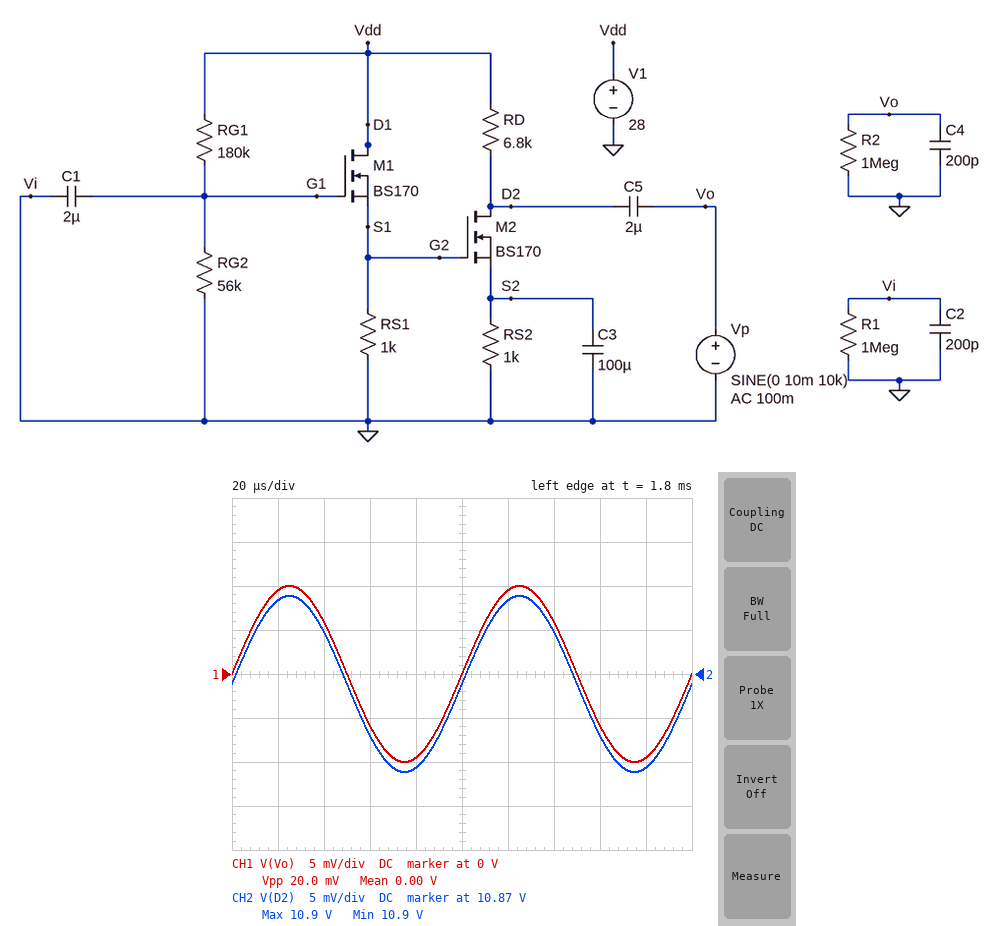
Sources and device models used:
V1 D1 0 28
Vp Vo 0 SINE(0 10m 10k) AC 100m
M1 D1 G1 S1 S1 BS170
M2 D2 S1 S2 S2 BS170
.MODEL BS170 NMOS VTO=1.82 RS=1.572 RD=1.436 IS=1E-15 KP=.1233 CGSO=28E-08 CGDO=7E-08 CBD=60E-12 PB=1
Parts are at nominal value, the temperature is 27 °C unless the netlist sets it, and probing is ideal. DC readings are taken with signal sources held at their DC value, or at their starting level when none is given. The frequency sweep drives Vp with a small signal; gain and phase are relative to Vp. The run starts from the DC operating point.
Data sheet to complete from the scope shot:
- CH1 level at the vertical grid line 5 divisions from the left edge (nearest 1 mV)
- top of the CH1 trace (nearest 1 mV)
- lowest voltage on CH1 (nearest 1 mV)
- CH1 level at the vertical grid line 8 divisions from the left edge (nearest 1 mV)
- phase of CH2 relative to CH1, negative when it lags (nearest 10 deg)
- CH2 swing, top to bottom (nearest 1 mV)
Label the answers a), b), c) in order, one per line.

a) 0 V
b) 10 mV
c) -10 mV
d) -6 mV
e) 0 deg
f) 20 mV
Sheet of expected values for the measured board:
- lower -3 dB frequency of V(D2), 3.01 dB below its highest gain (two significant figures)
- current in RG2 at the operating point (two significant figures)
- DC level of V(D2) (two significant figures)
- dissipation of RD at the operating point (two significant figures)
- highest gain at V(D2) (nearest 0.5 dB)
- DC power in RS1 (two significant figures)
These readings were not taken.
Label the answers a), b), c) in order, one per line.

a) 12 Hz
b) 120 µA
c) 11 V
d) 43 mW
e) 0 dB
f) 21 mW
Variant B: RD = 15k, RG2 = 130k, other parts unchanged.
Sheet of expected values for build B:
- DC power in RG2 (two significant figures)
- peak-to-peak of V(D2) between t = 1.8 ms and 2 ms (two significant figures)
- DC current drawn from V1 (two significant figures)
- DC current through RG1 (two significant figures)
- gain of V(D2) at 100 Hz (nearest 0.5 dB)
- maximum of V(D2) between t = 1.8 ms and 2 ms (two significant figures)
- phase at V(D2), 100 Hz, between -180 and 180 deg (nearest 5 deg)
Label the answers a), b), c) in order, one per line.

a) 1.1 mW
b) 9.5 mV
c) 11 mA
d) 90 µA
e) -34.0 dB
f) 1.8 V
g) 15 deg
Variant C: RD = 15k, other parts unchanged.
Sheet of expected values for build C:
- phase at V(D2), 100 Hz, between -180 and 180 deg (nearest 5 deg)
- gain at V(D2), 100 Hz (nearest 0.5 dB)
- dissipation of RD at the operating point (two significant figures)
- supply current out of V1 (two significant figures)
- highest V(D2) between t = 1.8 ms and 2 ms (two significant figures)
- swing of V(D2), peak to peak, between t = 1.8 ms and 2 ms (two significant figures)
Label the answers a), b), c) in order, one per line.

a) 35 deg
b) -32.0 dB
c) 46 mW
d) 6.4 mA
e) 1.8 V
f) 16 mV
